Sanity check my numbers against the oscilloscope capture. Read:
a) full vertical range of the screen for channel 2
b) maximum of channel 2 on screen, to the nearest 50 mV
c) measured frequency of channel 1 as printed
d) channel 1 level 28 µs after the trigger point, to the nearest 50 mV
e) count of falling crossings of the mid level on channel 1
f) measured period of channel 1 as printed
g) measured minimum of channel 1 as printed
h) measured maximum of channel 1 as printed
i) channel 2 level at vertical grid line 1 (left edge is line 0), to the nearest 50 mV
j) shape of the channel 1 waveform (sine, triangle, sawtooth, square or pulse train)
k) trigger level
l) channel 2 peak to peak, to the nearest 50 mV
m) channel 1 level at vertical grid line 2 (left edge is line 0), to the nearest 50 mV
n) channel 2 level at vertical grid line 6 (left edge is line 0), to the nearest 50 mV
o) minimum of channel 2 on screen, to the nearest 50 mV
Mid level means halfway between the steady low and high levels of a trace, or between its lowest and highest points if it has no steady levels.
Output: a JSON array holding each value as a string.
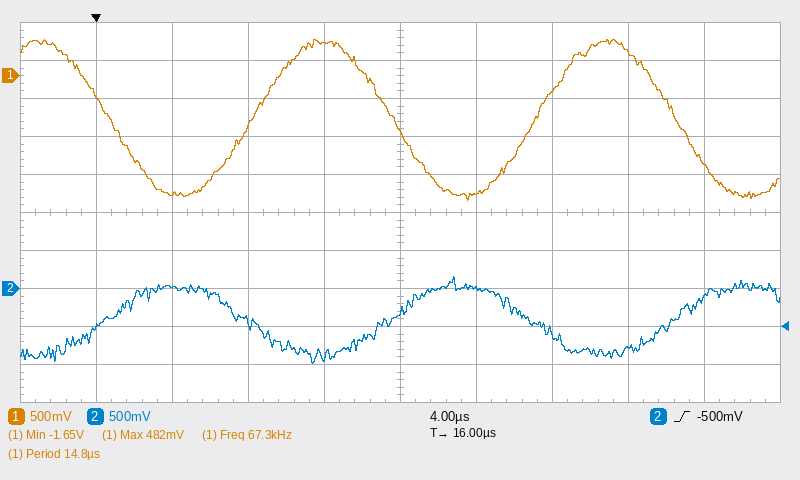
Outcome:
["5 V", "150 mV", "67.3 kHz", "300 mV", "3", "14.8 µs", "-1.65 V", "482 mV", "-500 mV", "sine", "-500 mV", "1.15 V", "-1.55 V", "0 mV", "-1.00 V"]
